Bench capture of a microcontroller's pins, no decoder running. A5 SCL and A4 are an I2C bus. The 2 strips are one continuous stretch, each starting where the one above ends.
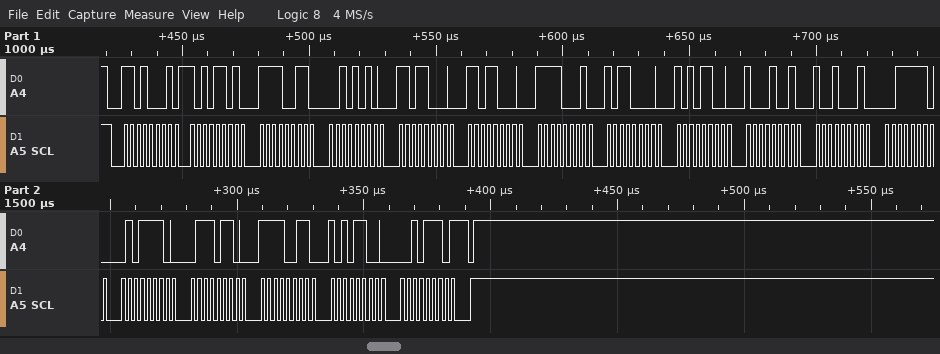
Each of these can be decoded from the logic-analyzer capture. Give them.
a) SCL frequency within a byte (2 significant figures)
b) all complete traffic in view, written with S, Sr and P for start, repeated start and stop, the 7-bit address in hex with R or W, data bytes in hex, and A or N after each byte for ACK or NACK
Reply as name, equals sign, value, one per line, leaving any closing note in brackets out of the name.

SCL frequency within a byte = 400 kHz
all complete traffic in view, written with S, Sr and P for start, repeated start and stop, the 7-bit address in hex with R or W, data bytes in hex, and A or N after each byte for ACK or NACK = S 68R A AD A F3 A 2A A D8 A D8 A F1 A B0 A AC A 89 A 91 A 3E A 5E A 76 A F3 A AC A 2E N P
